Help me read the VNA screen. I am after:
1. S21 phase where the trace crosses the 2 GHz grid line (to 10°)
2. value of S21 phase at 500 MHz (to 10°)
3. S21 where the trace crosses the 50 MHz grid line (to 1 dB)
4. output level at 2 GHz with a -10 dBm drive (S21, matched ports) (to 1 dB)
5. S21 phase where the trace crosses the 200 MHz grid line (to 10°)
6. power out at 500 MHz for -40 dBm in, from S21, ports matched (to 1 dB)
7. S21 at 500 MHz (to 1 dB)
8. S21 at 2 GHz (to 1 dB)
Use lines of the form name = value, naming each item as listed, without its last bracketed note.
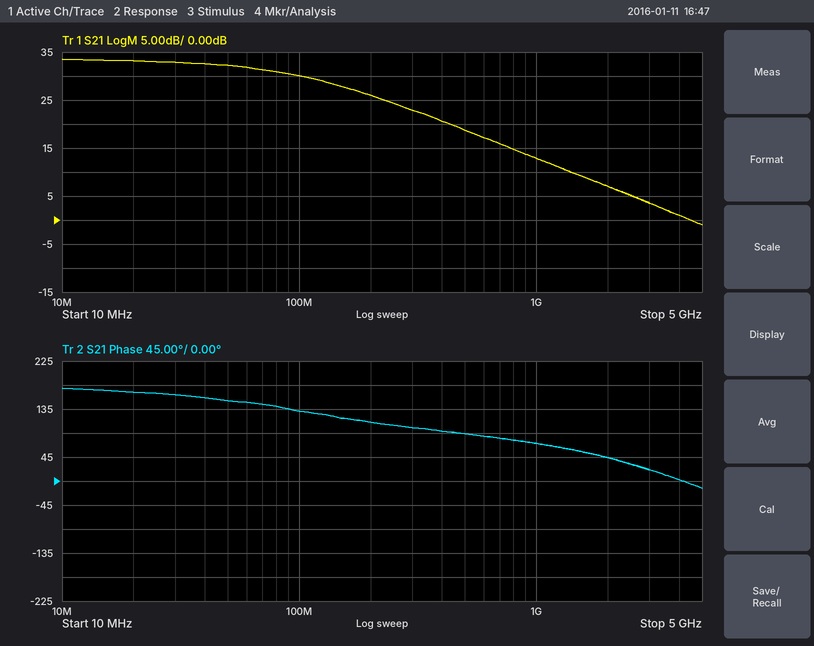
S21 phase where the trace crosses the 2 GHz grid line = 40°
value of S21 phase at 500 MHz = 90°
S21 where the trace crosses the 50 MHz grid line = 32 dB
output level at 2 GHz with a -10 dBm drive (S21, matched ports) = -3 dBm
S21 phase where the trace crosses the 200 MHz grid line = 110°
power out at 500 MHz for -40 dBm in, from S21, ports matched = -21 dBm
S21 at 500 MHz = 19 dB
S21 at 2 GHz = 7 dB
